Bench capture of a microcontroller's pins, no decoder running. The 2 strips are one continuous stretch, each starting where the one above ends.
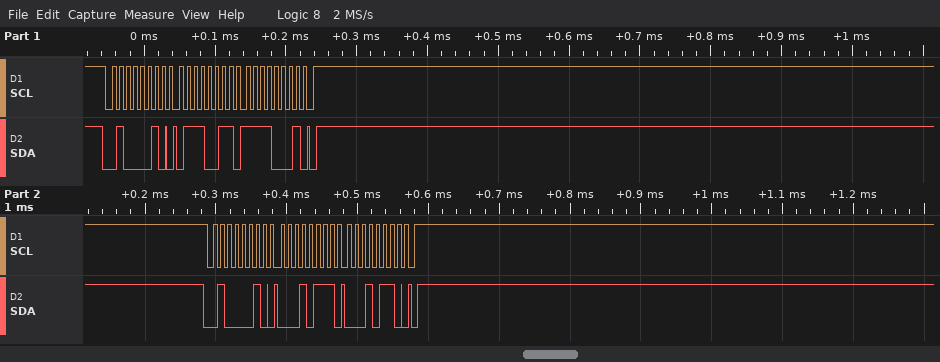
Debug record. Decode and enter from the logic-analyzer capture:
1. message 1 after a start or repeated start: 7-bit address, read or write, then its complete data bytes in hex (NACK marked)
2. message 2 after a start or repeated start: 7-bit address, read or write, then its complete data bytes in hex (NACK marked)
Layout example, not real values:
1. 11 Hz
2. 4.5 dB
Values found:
1. 0x21 write: 73 F1
2. 0x21 write: 17 16
